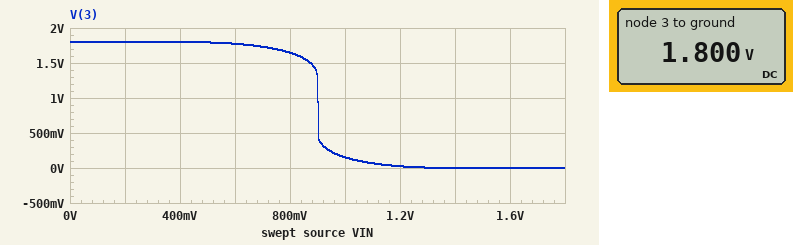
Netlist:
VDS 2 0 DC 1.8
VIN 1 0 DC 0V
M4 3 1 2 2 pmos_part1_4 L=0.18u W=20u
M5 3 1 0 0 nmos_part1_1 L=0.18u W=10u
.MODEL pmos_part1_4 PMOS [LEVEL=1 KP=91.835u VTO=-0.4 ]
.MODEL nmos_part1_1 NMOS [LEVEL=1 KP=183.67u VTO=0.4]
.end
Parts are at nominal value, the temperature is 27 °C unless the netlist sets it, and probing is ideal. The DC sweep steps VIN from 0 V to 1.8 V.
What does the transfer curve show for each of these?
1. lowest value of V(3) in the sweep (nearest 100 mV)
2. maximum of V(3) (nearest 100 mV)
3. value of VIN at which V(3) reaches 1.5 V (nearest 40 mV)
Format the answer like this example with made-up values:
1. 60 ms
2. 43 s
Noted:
1. 0 V
2. 1.8 V
3. 880 mV
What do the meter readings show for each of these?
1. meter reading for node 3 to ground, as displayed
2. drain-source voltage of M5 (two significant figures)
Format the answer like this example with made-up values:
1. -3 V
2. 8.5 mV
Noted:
1. 1.800 V
2. 1.8 V
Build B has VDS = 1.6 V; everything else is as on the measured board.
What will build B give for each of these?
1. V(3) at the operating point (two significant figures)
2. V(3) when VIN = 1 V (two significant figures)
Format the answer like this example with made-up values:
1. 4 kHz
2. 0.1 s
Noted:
1. 1.6 V
2. 34 mV
